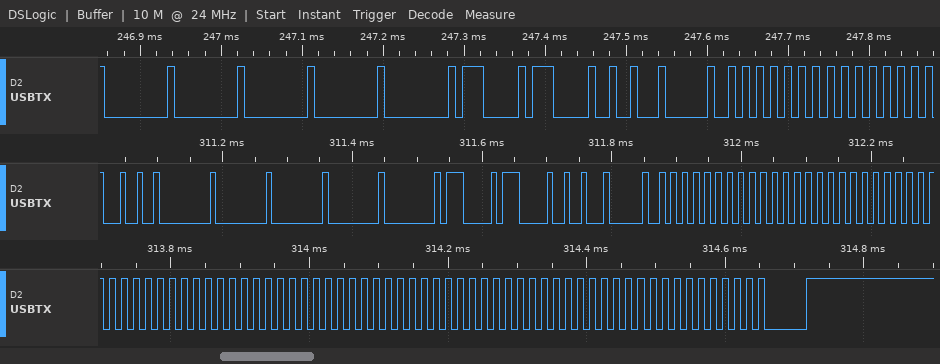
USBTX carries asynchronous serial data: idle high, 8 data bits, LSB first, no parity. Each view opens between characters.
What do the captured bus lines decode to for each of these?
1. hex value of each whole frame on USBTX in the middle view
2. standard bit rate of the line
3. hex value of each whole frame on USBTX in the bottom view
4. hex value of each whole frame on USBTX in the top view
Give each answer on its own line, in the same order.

24, 00, 00, 00, 00, 00, 07, 07, 12, 20, 55, 55, 55, 55
115200 baud
55, 55, 55, 55, 55, 55, 55, 55, 55, 55, 55, C0
00, 00, 00, 00, 00, 07, 07, 12, 20, 55, 55
